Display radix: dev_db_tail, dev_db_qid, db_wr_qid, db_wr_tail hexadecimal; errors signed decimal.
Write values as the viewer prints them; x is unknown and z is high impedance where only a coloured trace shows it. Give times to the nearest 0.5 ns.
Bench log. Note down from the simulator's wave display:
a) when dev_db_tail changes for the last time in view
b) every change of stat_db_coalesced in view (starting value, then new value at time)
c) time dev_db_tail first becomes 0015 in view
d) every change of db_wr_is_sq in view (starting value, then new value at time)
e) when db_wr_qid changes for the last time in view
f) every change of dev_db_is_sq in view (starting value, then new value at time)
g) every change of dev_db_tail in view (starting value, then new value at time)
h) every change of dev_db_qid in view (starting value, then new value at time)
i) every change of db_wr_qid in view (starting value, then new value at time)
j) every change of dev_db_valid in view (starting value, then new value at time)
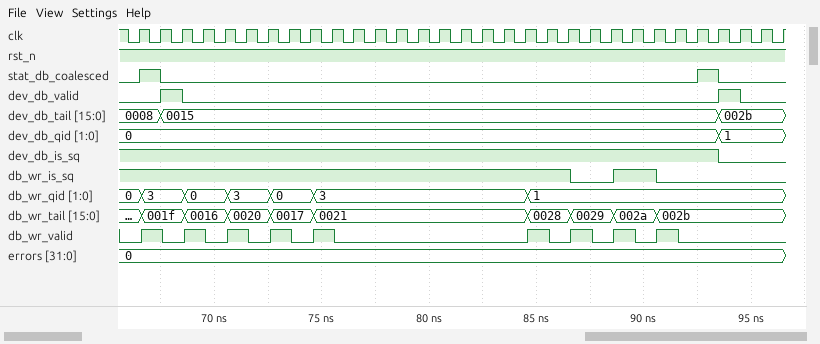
93.5 ns
0, 1 at 66.5 ns, 0 at 67.5 ns, 1 at 92.5 ns, 0 at 93.5 ns
67.5 ns
1, 0 at 86.5 ns, 1 at 88.5 ns, 0 at 90.5 ns
84.5 ns
1, 0 at 93.5 ns
0008, 0015 at 67.5 ns, 002b at 93.5 ns
0, 1 at 93.5 ns
0, 3 at 66.5 ns, 0 at 68.5 ns, 3 at 70.5 ns, 0 at 72.5 ns, 3 at 74.5 ns, 1 at 84.5 ns
0, 1 at 67.5 ns, 0 at 68.5 ns, 1 at 93.5 ns, 0 at 94.5 ns
